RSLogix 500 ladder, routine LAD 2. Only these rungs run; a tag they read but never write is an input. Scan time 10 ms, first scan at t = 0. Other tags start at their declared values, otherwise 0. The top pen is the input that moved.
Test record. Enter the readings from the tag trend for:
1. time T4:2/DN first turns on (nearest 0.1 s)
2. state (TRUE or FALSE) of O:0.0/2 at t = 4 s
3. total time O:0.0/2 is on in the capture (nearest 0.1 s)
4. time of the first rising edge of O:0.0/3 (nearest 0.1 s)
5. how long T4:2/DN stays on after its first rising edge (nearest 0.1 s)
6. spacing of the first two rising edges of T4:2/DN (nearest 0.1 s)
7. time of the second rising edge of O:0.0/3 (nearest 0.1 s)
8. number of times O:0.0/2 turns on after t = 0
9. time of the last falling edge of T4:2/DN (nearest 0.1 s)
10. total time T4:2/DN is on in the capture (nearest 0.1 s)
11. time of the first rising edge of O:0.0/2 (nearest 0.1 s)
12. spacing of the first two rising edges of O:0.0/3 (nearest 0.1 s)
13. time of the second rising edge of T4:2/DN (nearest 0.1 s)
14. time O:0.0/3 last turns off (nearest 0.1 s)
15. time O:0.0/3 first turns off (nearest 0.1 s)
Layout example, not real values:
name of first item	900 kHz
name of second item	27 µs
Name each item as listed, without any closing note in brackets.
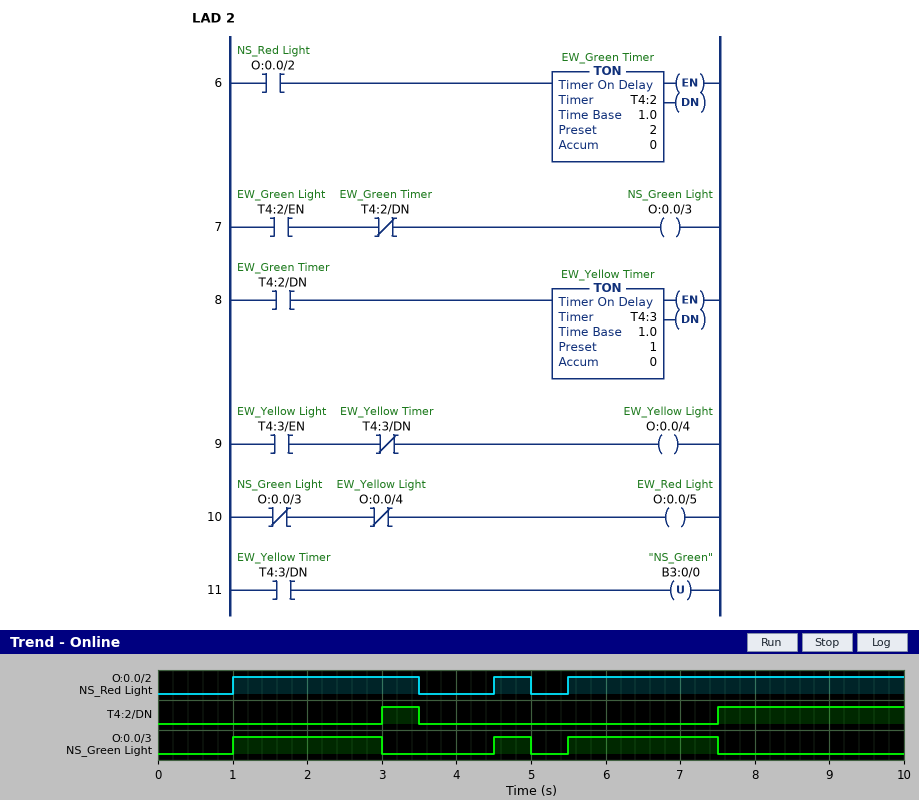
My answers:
time T4:2/DN first turns on	3.0 s
state (TRUE or FALSE) of O:0.0/2 at t = 4 s	FALSE
total time O:0.0/2 is on in the capture	7.5 s
time of the first rising edge of O:0.0/3	1.0 s
how long T4:2/DN stays on after its first rising edge	0.5 s
spacing of the first two rising edges of T4:2/DN	4.5 s
time of the second rising edge of O:0.0/3	4.5 s
number of times O:0.0/2 turns on after t = 0	3
time of the last falling edge of T4:2/DN	3.5 s
total time T4:2/DN is on in the capture	3.0 s
time of the first rising edge of O:0.0/2	1.0 s
spacing of the first two rising edges of O:0.0/3	3.5 s
time of the second rising edge of T4:2/DN	7.5 s
time O:0.0/3 last turns off	7.5 s
time O:0.0/3 first turns off	3.0 s
